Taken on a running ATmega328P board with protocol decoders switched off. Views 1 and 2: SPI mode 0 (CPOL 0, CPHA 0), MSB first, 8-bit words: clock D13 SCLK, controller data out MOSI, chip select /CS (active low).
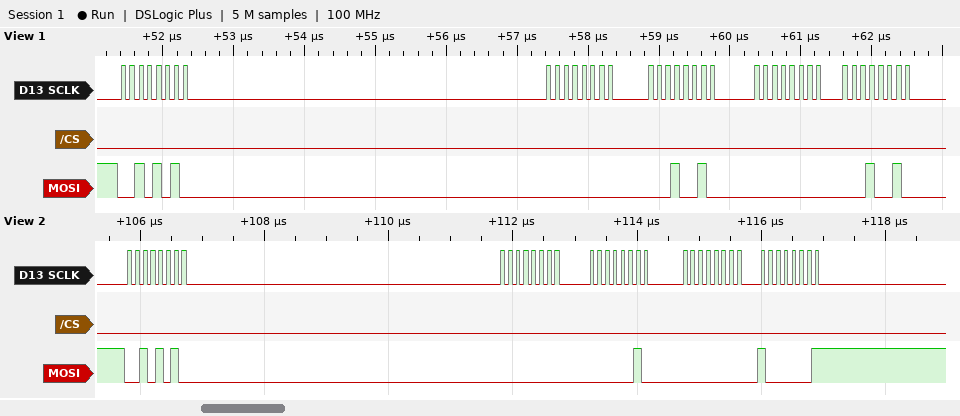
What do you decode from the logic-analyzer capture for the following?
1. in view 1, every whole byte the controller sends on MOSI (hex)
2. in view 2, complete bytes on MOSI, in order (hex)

0x2A 0x00 0x12 0x00 0x12
2A 00 02 00 81
